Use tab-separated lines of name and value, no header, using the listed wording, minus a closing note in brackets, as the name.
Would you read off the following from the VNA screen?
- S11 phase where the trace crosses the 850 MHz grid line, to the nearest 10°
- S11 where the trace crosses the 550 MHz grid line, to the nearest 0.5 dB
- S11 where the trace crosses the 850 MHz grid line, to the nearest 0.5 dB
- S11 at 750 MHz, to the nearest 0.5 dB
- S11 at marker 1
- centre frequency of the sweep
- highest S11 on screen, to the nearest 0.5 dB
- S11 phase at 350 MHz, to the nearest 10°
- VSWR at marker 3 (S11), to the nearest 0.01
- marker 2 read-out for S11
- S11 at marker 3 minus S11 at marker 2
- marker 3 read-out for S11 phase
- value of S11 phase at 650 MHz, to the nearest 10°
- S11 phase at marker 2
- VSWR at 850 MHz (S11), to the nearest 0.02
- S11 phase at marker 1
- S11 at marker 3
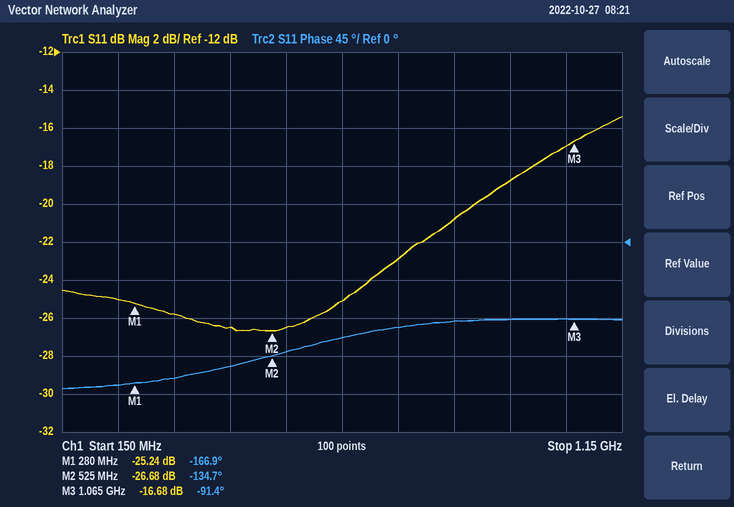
S11 phase where the trace crosses the 850 MHz grid line, to the nearest 10°	-90°
S11 where the trace crosses the 550 MHz grid line, to the nearest 0.5 dB	-26.5 dB
S11 where the trace crosses the 850 MHz grid line, to the nearest 0.5 dB	-21.0 dB
S11 at 750 MHz, to the nearest 0.5 dB	-23.0 dB
S11 at marker 1	-25.24 dB
centre frequency of the sweep	650 MHz
highest S11 on screen, to the nearest 0.5 dB	-15.5 dB
S11 phase at 350 MHz, to the nearest 10°	-160°
VSWR at marker 3 (S11), to the nearest 0.01	1.34
marker 2 read-out for S11	-26.68 dB
S11 at marker 3 minus S11 at marker 2	10.00 dB
marker 3 read-out for S11 phase	-91.4°
value of S11 phase at 650 MHz, to the nearest 10°	-110°
S11 phase at marker 2	-134.7°
VSWR at 850 MHz (S11), to the nearest 0.02	1.20
S11 phase at marker 1	-166.9°
S11 at marker 3	-16.68 dB
